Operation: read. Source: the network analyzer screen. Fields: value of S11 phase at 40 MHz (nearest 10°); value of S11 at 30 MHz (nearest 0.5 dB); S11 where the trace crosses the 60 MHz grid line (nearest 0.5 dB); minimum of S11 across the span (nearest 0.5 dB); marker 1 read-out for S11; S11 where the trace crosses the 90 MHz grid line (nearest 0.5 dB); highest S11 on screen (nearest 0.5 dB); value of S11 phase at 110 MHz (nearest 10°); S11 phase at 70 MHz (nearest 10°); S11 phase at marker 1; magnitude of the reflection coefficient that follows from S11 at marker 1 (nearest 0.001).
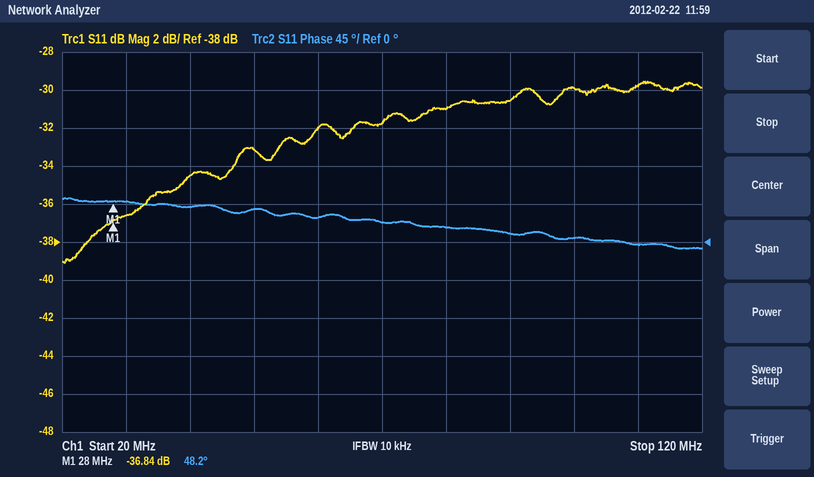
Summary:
40°
-36.5 dB
-32.0 dB
-39.0 dB
-36.84 dB
-30.5 dB
-29.5 dB
0°
20°
48.2°
0.014
